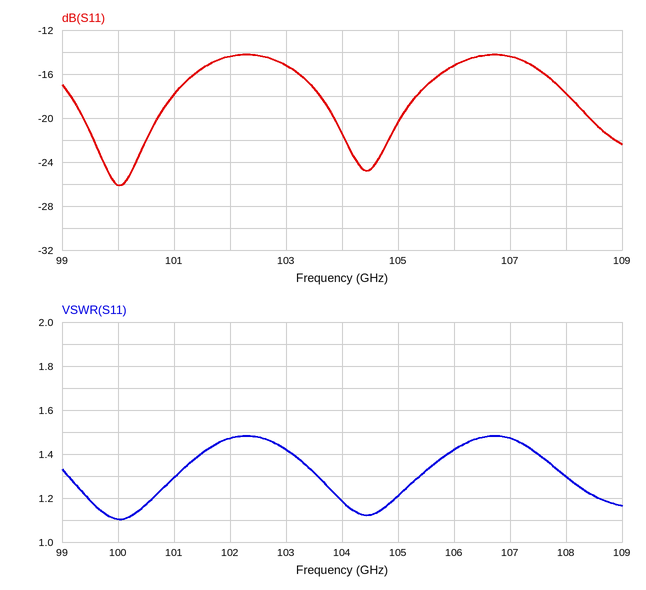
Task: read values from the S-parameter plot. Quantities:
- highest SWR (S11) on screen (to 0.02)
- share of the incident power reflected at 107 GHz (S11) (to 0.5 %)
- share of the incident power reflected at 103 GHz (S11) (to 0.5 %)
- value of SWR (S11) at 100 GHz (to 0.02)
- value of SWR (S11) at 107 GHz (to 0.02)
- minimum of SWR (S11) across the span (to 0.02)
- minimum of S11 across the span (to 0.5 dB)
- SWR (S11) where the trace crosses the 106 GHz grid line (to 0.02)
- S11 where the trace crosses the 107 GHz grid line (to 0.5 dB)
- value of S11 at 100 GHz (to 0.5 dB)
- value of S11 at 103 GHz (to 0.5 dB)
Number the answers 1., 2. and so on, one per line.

1. 1.48
2. 3.5 %
3. 3.0 %
4. 1.10
5. 1.48
6. 1.10
7. -26.0 dB
8. 1.42
9. -14.5 dB
10. -26.0 dB
11. -15.0 dB
